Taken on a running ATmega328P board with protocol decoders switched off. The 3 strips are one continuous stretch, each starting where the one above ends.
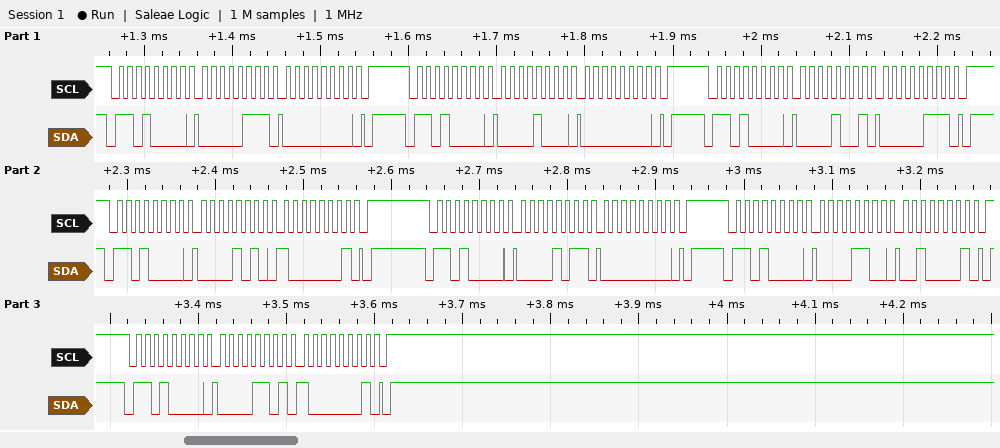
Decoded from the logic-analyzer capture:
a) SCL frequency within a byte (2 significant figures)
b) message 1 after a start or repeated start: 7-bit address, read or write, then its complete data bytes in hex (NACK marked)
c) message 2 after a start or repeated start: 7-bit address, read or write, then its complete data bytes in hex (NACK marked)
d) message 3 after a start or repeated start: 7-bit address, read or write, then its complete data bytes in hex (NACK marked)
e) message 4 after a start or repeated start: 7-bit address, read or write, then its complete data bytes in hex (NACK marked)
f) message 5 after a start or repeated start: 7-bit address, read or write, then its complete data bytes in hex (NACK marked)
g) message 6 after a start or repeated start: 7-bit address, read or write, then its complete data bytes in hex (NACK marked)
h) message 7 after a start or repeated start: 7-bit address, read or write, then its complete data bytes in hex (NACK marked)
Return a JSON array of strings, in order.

["100 kHz", "0x68 write: 07 00", "0x68 write: 08 00", "0x68 write: 09 07", "0x68 write: 0A 81", "0x68 write: 0B 00", "0x68 write: 0C 21", "0x68 write: 0D 81"]
